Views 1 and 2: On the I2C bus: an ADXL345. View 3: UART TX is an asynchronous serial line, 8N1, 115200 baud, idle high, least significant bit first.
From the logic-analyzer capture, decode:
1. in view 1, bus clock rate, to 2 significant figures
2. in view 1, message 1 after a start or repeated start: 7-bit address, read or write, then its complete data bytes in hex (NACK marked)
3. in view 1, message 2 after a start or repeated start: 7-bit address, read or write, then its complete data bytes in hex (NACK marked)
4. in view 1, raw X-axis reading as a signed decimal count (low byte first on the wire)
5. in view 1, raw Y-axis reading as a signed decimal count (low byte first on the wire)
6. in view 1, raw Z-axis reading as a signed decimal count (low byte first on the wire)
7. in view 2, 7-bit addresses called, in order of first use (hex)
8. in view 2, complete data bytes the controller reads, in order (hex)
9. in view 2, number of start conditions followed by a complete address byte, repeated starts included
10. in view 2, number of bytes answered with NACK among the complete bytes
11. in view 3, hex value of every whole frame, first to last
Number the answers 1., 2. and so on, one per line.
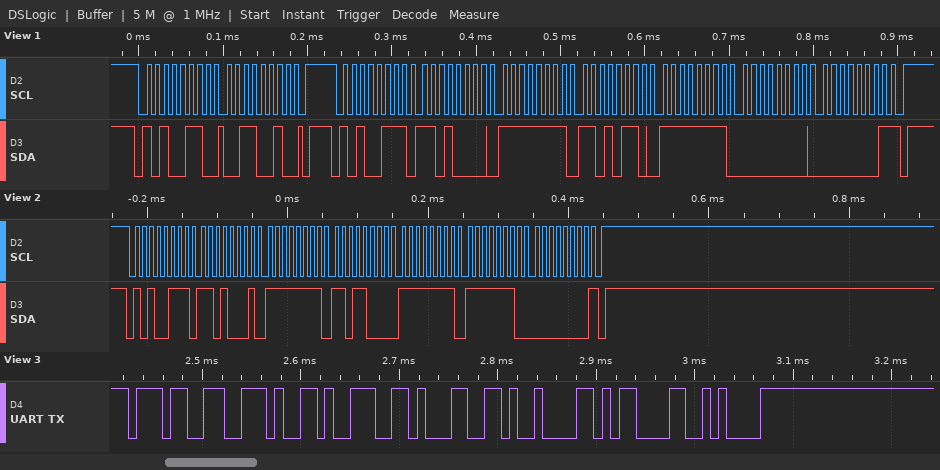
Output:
1. 100 kHz
2. 0x53 write: 32
3. 0x53 read: D0 FF D6 FF 00 01 NACK
4. -48
5. -42
6. 256
7. 0x53
8. D1 FF D8 FF FE 00
9. 1
10. 1
11. 37 2E 39 31 09 0D 0A
